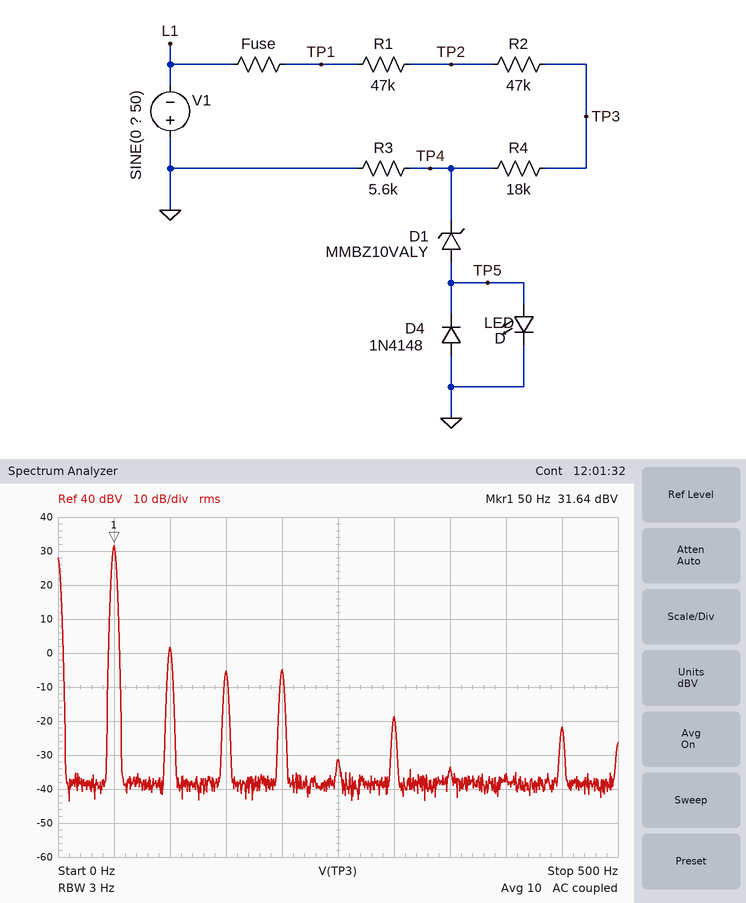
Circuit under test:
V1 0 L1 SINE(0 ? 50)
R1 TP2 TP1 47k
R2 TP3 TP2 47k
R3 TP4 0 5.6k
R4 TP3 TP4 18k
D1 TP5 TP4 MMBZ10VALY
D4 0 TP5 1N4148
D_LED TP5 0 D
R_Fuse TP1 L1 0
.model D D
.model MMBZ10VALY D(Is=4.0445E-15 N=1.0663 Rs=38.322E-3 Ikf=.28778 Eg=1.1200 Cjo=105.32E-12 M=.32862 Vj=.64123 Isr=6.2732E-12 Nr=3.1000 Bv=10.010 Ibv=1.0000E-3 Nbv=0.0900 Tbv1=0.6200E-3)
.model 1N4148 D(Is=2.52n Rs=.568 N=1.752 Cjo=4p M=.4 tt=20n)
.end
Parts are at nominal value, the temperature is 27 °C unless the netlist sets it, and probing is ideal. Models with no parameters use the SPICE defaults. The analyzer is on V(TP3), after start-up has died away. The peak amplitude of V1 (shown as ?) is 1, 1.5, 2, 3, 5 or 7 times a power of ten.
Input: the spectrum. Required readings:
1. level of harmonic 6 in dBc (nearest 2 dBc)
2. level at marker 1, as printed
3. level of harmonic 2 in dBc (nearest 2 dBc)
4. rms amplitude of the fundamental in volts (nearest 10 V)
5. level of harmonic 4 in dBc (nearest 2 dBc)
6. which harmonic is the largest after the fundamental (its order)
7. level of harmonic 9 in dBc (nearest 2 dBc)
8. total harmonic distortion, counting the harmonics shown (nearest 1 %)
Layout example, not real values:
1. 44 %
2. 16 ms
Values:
1. -50 dBc
2. 31.64 dBV
3. -30 dBc
4. 40 V
5. -36 dBc
6. 2
7. -54 dBc
8. 4 %
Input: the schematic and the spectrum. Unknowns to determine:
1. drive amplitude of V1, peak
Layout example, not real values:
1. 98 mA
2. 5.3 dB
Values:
1. 300 V
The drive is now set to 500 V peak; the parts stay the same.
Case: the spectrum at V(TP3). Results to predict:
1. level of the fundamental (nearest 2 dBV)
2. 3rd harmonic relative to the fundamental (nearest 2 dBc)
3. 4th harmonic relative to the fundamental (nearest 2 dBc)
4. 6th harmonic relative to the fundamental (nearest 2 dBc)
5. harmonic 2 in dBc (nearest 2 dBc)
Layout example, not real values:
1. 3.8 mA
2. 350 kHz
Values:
1. 36 dBV
2. -34 dBc
3. -40 dBc
4. -42 dBc
5. -38 dBc
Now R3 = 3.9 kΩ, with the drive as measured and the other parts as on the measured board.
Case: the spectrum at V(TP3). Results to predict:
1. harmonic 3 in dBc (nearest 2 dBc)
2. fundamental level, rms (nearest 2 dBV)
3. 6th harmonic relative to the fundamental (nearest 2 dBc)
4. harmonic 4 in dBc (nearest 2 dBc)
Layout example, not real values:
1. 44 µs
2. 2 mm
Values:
1. -48 dBc
2. 32 dBV
3. -54 dBc
4. -44 dBc
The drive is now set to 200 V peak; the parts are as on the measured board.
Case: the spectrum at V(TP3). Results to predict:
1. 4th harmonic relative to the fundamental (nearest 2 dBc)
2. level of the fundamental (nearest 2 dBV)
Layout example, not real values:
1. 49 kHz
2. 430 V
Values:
1. -42 dBc
2. 28 dBV
